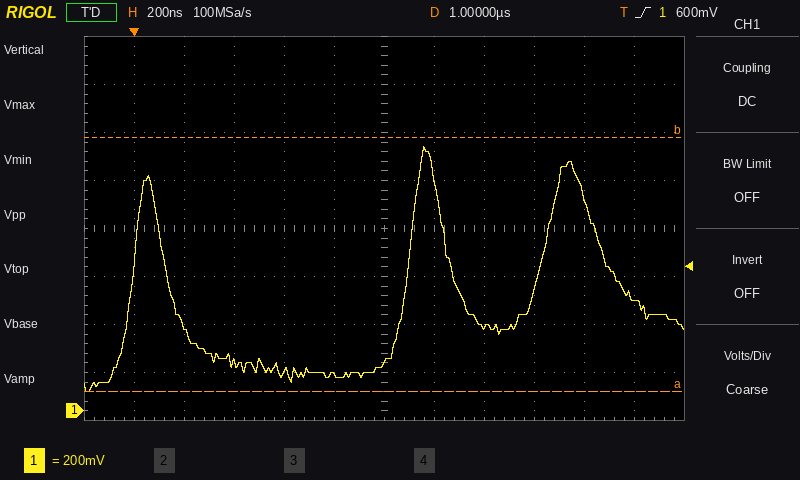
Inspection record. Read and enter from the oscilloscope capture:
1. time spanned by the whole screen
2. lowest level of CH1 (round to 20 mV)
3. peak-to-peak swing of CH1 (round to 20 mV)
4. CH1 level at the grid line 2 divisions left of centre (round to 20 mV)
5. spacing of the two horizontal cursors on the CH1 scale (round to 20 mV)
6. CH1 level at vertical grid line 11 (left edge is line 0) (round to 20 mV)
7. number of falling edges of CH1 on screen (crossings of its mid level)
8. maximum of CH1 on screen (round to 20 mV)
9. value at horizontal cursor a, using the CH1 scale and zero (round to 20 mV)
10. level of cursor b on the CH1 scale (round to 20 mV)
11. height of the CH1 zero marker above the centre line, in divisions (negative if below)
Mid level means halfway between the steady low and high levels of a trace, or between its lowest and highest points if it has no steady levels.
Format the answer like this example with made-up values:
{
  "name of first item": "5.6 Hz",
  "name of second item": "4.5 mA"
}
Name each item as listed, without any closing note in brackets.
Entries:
{
  "time spanned by the whole screen": "2.4 µs",
  "lowest level of CH1": "80 mV",
  "peak-to-peak swing of CH1": "1.02 V",
  "CH1 level at the grid line 2 divisions left of centre": "160 mV",
  "spacing of the two horizontal cursors on the CH1 scale": "1.06 V",
  "CH1 level at vertical grid line 11 (left edge is line 0)": "460 mV",
  "number of falling edges of CH1 on screen": "3",
  "maximum of CH1 on screen": "1.10 V",
  "value at horizontal cursor a, using the CH1 scale and zero": "80 mV",
  "level of cursor b on the CH1 scale": "1.14 V",
  "height of the CH1 zero marker above the centre line, in divisions": "-3.8 div"
}
